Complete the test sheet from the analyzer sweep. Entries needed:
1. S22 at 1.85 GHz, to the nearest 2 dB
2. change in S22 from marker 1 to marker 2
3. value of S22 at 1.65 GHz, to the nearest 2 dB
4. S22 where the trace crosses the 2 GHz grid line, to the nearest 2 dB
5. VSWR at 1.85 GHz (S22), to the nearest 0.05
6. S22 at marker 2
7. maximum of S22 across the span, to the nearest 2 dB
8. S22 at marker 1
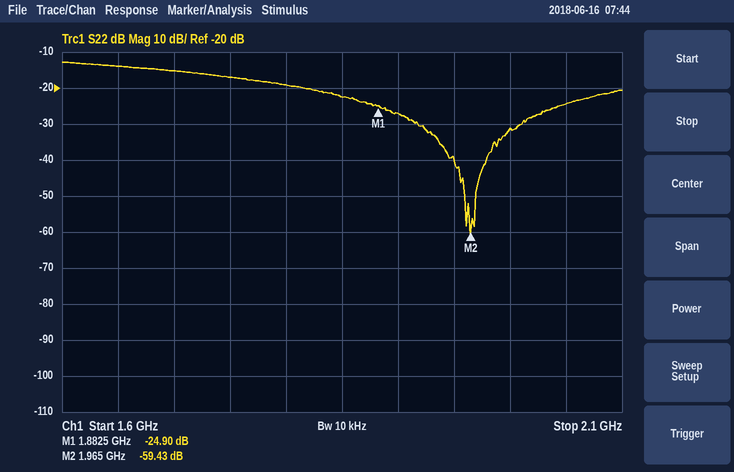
-22 dB
-34.53 dB
-14 dB
-32 dB
1.15
-59.43 dB
-12 dB
-24.90 dB
